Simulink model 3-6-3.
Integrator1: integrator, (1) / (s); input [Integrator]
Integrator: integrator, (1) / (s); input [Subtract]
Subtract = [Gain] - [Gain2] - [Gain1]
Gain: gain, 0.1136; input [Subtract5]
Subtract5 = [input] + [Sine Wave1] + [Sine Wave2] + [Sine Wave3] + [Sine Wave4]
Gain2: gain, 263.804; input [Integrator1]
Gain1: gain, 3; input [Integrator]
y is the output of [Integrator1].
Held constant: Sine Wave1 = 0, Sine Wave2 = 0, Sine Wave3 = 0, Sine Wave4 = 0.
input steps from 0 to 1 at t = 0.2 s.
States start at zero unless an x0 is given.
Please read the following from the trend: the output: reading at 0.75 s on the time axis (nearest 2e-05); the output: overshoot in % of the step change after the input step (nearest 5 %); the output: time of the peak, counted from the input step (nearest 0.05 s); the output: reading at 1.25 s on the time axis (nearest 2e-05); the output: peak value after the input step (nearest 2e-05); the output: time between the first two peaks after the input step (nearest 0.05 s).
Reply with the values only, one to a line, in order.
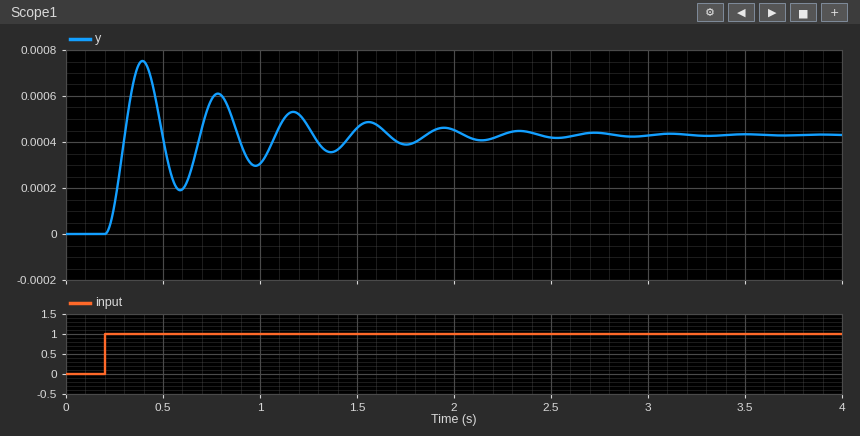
0.00058
75 %
0.20 s
0.00046
0.00076
0.40 s
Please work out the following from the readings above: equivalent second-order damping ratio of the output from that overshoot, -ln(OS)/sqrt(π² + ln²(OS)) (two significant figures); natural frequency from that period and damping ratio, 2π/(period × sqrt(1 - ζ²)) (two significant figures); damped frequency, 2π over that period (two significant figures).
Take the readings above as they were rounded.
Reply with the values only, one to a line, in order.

0.091
16 rad/s
16 rad/s
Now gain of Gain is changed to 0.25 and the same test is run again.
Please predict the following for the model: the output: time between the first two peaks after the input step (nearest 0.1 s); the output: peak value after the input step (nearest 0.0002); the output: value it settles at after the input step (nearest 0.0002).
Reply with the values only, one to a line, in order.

0.4 s
0.0016
0.0010
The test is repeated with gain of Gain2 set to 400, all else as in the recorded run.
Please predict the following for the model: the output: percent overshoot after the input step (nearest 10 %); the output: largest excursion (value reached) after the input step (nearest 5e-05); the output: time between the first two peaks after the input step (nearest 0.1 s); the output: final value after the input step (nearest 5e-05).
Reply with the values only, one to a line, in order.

80 %
0.00050
0.3 s
0.00030
